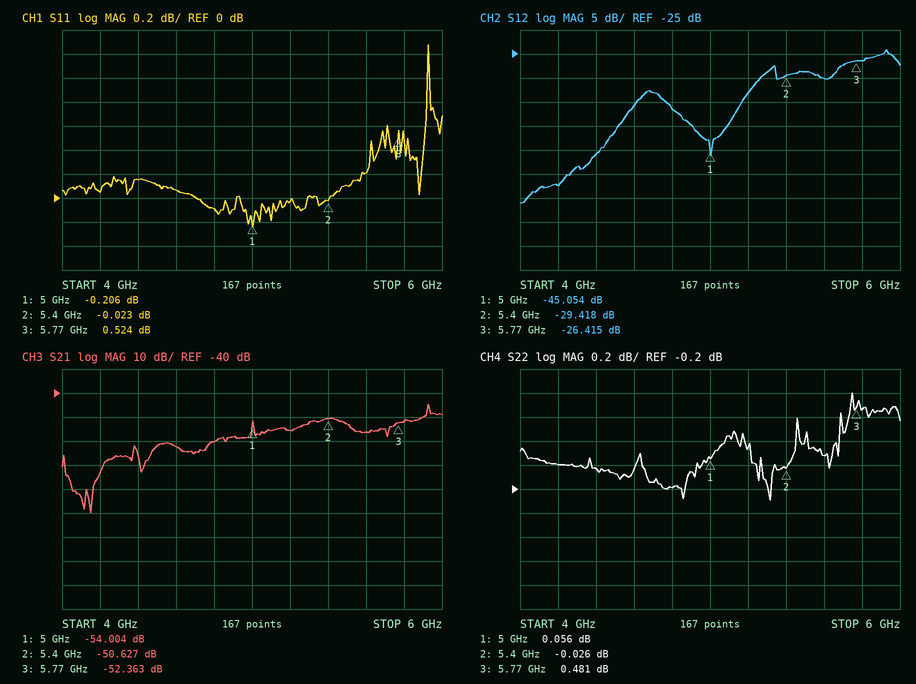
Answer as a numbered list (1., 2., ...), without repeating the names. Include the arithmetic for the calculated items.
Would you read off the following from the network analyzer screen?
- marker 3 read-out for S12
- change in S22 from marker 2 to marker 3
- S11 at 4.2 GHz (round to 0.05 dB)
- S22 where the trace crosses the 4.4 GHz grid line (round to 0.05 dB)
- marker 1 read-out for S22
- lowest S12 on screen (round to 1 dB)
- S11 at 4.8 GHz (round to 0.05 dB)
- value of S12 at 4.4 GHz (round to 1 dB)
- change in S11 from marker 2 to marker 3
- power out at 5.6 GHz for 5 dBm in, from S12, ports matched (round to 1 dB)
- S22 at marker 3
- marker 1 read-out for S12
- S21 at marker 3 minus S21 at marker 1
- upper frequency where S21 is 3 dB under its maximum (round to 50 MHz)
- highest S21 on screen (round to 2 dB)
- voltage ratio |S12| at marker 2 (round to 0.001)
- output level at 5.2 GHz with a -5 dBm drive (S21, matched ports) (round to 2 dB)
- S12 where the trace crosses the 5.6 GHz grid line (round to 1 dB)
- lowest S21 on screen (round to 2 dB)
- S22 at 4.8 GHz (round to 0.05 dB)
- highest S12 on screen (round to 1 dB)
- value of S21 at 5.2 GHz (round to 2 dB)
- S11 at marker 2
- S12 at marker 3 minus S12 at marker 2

1. -26.415 dB
2. 0.481 − (-0.026) = 0.507 dB
3. 0.05 dB
4. -0.05 dB
5. 0.056 dB
6. -56 dB
7. -0.10 dB
8. -46 dB
9. 0.524 − (-0.023) = 0.547 dB
10. 5 dBm + (-30 dB) = -25 dBm
11. 0.481 dB
12. -45.054 dB
13. -52.363 − (-54.004) = 1.641 dB
14. 5.95 GHz
15. -44 dB
16. 10^(-29.418/20) ≈ 0.034
17. -5 dBm + (-56 dB) = -60 dBm
18. -30 dB
19. -90 dB
20. -0.20 dB
21. -24 dB
22. -56 dB
23. -0.023 dB
24. -26.415 − (-29.418) = 3.003 dB
